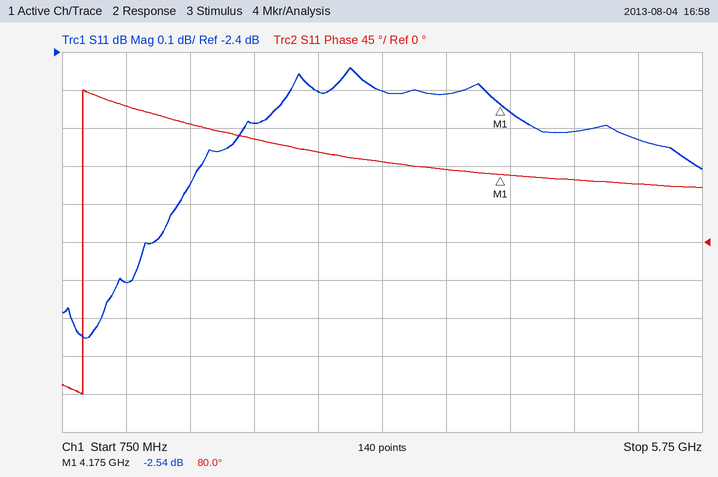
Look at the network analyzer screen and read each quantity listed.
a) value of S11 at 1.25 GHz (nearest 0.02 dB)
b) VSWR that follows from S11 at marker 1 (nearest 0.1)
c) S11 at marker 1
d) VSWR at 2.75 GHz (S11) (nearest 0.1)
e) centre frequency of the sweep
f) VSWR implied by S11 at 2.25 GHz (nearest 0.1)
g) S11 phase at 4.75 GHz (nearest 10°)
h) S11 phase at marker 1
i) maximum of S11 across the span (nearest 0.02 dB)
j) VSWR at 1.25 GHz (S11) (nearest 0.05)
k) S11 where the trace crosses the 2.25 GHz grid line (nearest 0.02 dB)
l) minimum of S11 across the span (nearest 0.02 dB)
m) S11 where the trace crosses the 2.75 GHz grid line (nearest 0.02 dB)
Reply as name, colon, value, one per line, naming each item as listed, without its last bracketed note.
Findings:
value of S11 at 1.25 GHz: -3.00 dB
VSWR that follows from S11 at marker 1: 6.9
S11 at marker 1: -2.54 dB
VSWR at 2.75 GHz (S11): 7.0
centre frequency of the sweep: 3.25 GHz
VSWR implied by S11 at 2.25 GHz: 6.8
S11 phase at 4.75 GHz: 70°
S11 phase at marker 1: 80.0°
maximum of S11 across the span: -2.44 dB
VSWR at 1.25 GHz (S11): 5.85
S11 where the trace crosses the 2.25 GHz grid line: -2.58 dB
minimum of S11 across the span: -3.16 dB
S11 where the trace crosses the 2.75 GHz grid line: -2.50 dB
